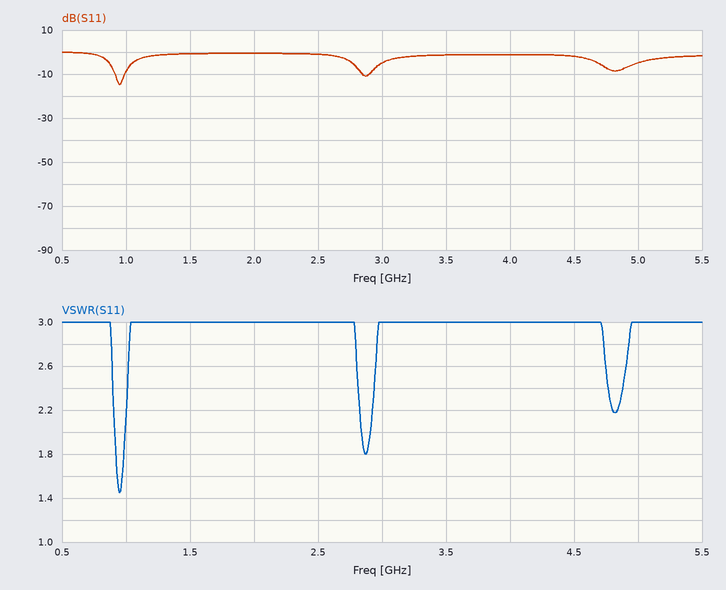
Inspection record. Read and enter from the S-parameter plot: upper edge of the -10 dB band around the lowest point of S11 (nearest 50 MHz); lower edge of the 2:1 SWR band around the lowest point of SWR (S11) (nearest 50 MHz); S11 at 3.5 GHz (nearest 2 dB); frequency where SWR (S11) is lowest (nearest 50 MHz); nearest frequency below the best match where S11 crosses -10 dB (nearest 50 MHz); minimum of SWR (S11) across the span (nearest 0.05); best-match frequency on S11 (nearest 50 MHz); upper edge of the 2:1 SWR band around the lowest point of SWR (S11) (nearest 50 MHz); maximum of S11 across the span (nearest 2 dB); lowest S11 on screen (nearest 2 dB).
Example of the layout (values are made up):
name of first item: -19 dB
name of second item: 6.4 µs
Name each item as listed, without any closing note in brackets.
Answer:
upper edge of the -10 dB band around the lowest point of S11: 1.00 GHz
lower edge of the 2:1 SWR band around the lowest point of SWR (S11): 900 MHz
S11 at 3.5 GHz: -2 dB
frequency where SWR (S11) is lowest: 950 MHz
nearest frequency below the best match where S11 crosses -10 dB: 900 MHz
minimum of SWR (S11) across the span: 1.45
best-match frequency on S11: 950 MHz
upper edge of the 2:1 SWR band around the lowest point of SWR (S11): 1.00 GHz
maximum of S11 across the span: 0 dB
lowest S11 on screen: -14 dB
